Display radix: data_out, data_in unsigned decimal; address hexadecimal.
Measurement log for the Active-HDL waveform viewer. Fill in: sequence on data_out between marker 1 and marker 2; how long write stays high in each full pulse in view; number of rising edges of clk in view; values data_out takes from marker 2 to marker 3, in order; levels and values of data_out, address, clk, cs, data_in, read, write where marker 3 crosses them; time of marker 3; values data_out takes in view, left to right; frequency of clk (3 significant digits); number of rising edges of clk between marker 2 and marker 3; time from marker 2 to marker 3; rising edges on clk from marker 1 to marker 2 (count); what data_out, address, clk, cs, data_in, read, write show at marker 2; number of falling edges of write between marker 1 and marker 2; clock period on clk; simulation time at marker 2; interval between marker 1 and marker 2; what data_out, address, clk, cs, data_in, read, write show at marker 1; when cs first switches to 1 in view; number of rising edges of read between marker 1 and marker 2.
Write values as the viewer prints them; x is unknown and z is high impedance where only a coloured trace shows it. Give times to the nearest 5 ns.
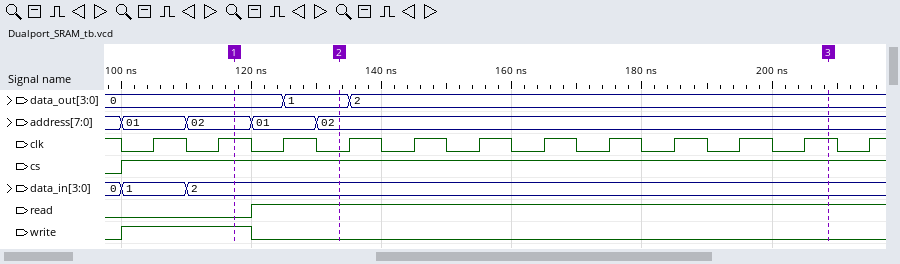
0, 1
20 ns
12
1, 2
data_out=2, address=02, clk=1, cs=1, data_in=2, read=1, write=0
210 ns
0, 1, 2
100 MHz
8
75 ns
1
data_out=1, address=02, clk=0, cs=1, data_in=2, read=1, write=0
1
10 ns
135 ns
15 ns
data_out=0, address=02, clk=1, cs=1, data_in=2, read=0, write=1
100 ns
1
